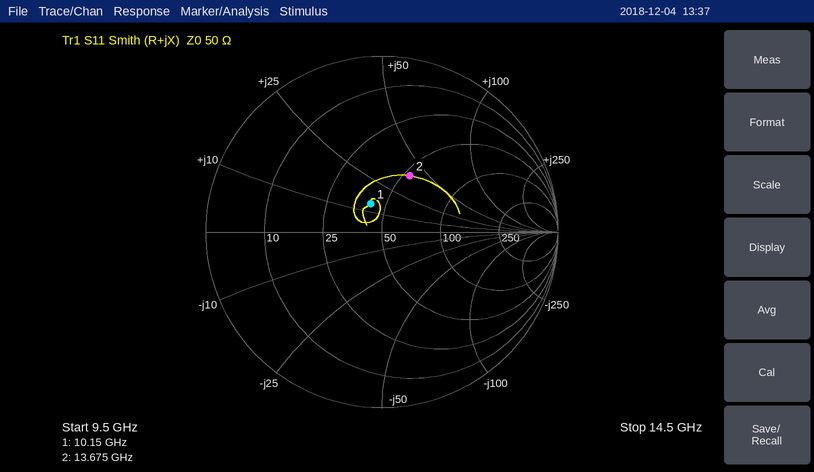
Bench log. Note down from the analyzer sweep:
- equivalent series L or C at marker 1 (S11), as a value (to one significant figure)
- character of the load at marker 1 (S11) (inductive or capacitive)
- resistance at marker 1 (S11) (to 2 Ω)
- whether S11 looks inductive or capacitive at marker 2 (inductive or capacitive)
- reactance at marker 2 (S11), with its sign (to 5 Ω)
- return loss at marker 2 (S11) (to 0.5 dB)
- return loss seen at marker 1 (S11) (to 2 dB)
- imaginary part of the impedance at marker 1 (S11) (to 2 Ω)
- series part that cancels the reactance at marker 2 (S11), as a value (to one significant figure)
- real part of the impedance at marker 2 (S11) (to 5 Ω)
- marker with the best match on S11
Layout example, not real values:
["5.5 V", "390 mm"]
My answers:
["200 pH", "inductive", "42 Ω", "inductive", "+40 Ω", "9.0 dB", "16 dB", "+14 Ω", "300 fF", "55 Ω", "marker 1"]
